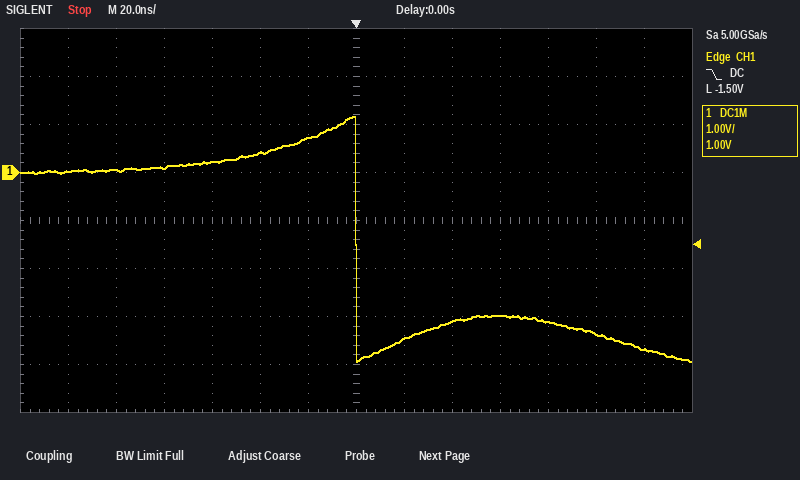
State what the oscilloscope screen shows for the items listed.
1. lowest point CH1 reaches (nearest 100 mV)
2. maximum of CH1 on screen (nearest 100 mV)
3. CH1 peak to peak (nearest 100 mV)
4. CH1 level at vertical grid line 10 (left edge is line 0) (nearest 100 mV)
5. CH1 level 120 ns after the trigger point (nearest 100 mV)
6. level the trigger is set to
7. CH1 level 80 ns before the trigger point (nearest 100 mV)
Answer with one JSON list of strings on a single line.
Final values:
["-3.9 V", "1.2 V", "5.1 V", "-3.0 V", "-3.7 V", "-1.50 V", "100 mV"]
